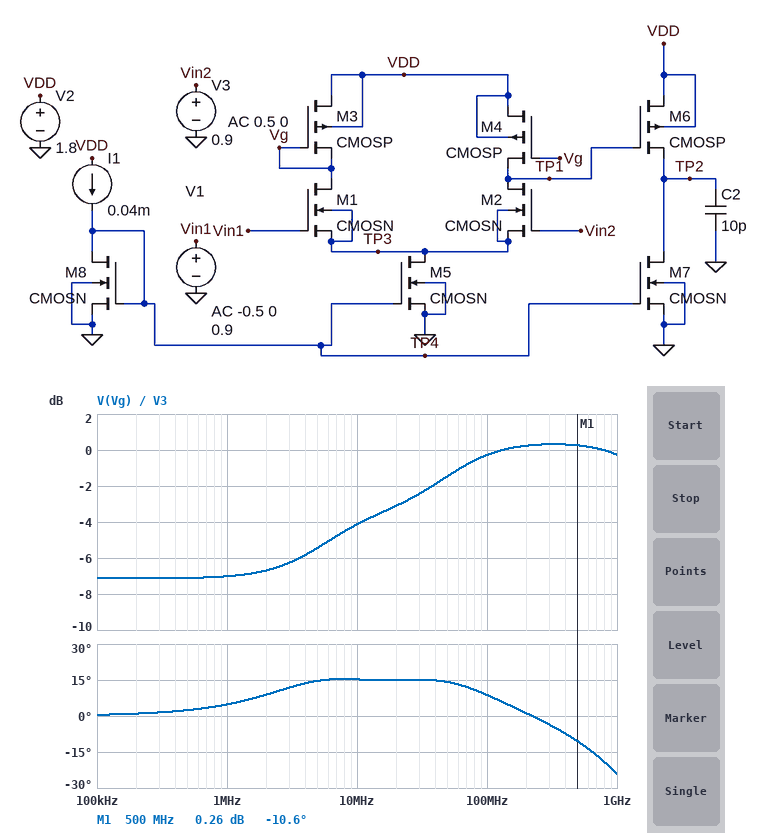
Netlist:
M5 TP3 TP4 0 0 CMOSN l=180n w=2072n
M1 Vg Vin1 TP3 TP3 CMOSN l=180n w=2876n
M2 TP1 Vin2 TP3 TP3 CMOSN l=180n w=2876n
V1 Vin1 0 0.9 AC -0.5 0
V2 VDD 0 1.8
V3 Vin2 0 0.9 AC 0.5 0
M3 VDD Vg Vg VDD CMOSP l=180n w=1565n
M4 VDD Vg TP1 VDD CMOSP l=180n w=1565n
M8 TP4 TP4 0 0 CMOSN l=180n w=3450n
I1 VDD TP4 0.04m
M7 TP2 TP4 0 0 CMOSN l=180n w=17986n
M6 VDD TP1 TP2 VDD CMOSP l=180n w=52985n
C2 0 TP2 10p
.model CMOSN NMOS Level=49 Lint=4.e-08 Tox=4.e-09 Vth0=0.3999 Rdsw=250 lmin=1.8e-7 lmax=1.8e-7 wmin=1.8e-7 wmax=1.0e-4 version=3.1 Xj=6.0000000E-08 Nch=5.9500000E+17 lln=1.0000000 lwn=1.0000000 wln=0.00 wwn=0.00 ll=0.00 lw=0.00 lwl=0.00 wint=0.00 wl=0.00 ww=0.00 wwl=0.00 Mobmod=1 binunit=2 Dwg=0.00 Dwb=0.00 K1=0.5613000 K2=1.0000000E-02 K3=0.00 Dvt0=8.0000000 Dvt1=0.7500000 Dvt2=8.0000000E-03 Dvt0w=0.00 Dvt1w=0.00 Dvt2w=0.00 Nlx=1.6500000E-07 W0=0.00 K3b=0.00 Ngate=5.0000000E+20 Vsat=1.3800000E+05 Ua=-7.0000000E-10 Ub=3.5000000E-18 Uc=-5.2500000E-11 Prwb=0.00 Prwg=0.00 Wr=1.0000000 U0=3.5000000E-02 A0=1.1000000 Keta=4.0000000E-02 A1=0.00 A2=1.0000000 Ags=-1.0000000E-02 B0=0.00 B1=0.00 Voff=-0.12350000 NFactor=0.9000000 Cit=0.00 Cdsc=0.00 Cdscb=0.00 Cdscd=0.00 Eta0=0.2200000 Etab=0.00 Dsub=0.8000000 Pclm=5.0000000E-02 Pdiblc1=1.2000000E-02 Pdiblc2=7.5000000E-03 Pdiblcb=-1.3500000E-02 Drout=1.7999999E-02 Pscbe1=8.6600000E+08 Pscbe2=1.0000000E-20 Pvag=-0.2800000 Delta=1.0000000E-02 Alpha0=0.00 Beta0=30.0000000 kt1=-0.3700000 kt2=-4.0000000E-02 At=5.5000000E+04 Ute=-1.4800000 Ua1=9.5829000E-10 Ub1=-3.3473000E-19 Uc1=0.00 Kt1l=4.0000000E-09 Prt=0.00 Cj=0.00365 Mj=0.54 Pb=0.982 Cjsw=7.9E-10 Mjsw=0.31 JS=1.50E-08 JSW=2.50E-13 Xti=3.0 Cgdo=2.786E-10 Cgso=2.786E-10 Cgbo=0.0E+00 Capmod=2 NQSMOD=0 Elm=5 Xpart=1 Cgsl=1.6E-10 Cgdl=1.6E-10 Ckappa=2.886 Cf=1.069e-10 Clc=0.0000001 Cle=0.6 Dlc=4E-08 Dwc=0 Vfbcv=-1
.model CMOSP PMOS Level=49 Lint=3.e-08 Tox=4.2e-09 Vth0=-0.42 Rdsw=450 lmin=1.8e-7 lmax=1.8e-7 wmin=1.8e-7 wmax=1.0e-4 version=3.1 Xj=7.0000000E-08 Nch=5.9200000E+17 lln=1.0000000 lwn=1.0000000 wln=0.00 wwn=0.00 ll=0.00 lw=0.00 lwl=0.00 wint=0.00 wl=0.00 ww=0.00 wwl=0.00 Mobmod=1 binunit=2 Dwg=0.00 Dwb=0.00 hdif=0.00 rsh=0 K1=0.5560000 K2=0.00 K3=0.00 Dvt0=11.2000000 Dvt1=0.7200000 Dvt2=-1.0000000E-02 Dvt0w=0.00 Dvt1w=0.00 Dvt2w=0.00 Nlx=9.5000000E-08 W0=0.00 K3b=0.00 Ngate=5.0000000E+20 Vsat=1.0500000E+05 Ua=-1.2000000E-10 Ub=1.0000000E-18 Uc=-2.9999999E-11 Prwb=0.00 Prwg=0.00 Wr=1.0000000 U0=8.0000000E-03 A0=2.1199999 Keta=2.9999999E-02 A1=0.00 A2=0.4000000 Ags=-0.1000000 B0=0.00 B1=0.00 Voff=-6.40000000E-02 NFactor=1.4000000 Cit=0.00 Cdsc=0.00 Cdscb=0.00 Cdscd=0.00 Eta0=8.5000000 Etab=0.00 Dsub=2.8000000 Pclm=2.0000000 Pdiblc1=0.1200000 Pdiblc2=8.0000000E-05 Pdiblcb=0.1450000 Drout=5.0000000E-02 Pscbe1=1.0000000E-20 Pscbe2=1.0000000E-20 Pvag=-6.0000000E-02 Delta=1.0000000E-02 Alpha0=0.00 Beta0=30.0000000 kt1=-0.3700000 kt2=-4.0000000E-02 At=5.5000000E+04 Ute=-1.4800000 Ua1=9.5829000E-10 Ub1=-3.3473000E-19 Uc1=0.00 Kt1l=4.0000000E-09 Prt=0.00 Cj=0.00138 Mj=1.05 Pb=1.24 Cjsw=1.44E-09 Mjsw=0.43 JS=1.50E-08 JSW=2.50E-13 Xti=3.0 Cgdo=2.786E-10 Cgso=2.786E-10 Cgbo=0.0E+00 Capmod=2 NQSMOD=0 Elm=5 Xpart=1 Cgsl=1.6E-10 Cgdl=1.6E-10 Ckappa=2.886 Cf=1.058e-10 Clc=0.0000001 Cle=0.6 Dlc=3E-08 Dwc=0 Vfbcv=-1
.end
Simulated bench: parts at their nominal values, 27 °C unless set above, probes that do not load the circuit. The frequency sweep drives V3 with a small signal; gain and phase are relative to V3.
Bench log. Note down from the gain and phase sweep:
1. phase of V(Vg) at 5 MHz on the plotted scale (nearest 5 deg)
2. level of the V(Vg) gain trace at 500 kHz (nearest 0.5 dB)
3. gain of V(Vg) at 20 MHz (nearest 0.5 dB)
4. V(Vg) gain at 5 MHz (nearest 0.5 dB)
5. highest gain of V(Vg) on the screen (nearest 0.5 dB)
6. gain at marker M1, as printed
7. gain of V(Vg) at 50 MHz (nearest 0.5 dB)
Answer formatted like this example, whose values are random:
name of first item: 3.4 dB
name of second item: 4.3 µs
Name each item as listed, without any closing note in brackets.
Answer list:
phase of V(Vg) at 5 MHz on the plotted scale: 15 deg
level of the V(Vg) gain trace at 500 kHz: -7.0 dB
gain of V(Vg) at 20 MHz: -3.0 dB
V(Vg) gain at 5 MHz: -5.5 dB
highest gain of V(Vg) on the screen: 0.5 dB
gain at marker M1, as printed: 0.26 dB
gain of V(Vg) at 50 MHz: -1.5 dB
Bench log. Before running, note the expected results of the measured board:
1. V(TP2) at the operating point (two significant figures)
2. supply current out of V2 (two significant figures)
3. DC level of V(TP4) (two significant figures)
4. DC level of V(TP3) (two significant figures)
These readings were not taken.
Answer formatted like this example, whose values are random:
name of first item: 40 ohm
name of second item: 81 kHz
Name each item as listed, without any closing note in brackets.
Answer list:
V(TP2) at the operating point: 1.3 V
supply current out of V2: 520 µA
DC level of V(TP4): 480 mV
DC level of V(TP3): 510 mV
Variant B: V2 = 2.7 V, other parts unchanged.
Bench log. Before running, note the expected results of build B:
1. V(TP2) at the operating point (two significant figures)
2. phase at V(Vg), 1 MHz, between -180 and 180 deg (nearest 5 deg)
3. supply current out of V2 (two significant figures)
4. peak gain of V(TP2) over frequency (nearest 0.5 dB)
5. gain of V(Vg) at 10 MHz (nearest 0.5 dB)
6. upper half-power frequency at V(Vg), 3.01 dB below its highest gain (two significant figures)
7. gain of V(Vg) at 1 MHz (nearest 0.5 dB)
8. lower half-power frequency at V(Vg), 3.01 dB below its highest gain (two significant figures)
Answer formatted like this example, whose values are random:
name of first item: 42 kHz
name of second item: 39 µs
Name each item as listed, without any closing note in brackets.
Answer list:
V(TP2) at the operating point: 1.7 V
phase at V(Vg), 1 MHz, between -180 and 180 deg: 5 deg
supply current out of V2: 710 µA
peak gain of V(TP2) over frequency: 40.0 dB
gain of V(Vg) at 10 MHz: -3.5 dB
upper half-power frequency at V(Vg), 3.01 dB below its highest gain: 2.5 GHz
gain of V(Vg) at 1 MHz: -6.5 dB
lower half-power frequency at V(Vg), 3.01 dB below its highest gain: 25 MHz
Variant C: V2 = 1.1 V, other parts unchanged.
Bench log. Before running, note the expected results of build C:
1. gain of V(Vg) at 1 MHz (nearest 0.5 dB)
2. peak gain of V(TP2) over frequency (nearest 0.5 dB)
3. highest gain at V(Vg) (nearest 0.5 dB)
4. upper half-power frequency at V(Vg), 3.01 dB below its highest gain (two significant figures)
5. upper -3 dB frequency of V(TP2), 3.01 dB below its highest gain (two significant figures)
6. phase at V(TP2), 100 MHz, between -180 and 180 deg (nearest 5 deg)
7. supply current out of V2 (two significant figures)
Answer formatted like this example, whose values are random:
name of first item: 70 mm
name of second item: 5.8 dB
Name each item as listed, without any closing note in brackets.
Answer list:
gain of V(Vg) at 1 MHz: -8.0 dB
peak gain of V(TP2) over frequency: 35.0 dB
highest gain at V(Vg): 0 dB
upper half-power frequency at V(Vg), 3.01 dB below its highest gain: 2.3 GHz
upper -3 dB frequency of V(TP2), 3.01 dB below its highest gain: 7.3 MHz
phase at V(TP2), 100 MHz, between -180 and 180 deg: -150 deg
supply current out of V2: 390 µA
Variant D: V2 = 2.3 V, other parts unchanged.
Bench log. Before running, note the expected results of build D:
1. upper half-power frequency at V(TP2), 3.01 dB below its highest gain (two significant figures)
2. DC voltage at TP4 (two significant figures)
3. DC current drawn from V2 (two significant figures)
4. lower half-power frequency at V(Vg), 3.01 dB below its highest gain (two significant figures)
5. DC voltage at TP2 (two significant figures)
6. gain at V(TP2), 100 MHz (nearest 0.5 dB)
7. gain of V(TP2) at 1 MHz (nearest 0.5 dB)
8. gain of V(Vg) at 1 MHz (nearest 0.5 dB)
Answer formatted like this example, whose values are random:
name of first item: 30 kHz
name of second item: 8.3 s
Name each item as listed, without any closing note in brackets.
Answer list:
upper half-power frequency at V(TP2), 3.01 dB below its highest gain: 7.0 MHz
DC voltage at TP4: 480 mV
DC current drawn from V2: 620 µA
lower half-power frequency at V(Vg), 3.01 dB below its highest gain: 25 MHz
DC voltage at TP2: 1.5 V
gain at V(TP2), 100 MHz: 11.0 dB
gain of V(TP2) at 1 MHz: 39.0 dB
gain of V(Vg) at 1 MHz: -6.5 dB
